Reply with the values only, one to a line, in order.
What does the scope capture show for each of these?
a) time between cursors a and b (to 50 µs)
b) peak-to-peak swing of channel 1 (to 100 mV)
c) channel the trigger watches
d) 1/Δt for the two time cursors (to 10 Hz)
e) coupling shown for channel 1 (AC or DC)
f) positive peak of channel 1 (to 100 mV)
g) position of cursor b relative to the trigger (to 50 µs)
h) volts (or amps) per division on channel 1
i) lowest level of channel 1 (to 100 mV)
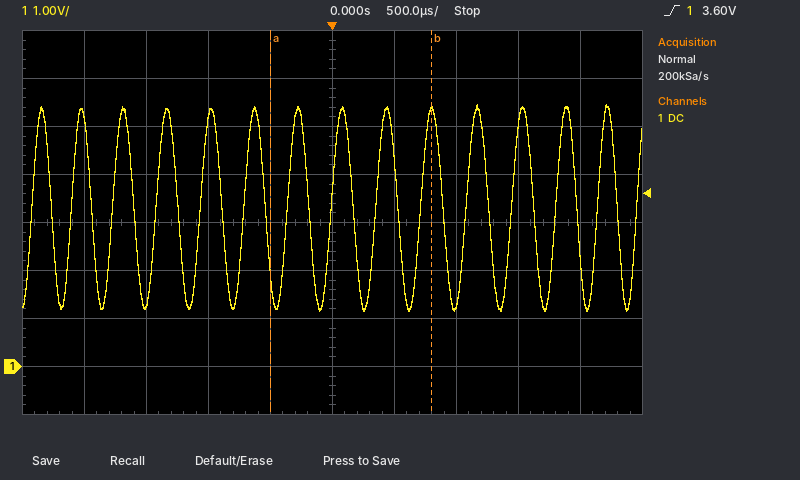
1.30 ms
4.3 V
channel 1
770 Hz
DC
5.5 V
+800 µs
1 V
1.2 V
